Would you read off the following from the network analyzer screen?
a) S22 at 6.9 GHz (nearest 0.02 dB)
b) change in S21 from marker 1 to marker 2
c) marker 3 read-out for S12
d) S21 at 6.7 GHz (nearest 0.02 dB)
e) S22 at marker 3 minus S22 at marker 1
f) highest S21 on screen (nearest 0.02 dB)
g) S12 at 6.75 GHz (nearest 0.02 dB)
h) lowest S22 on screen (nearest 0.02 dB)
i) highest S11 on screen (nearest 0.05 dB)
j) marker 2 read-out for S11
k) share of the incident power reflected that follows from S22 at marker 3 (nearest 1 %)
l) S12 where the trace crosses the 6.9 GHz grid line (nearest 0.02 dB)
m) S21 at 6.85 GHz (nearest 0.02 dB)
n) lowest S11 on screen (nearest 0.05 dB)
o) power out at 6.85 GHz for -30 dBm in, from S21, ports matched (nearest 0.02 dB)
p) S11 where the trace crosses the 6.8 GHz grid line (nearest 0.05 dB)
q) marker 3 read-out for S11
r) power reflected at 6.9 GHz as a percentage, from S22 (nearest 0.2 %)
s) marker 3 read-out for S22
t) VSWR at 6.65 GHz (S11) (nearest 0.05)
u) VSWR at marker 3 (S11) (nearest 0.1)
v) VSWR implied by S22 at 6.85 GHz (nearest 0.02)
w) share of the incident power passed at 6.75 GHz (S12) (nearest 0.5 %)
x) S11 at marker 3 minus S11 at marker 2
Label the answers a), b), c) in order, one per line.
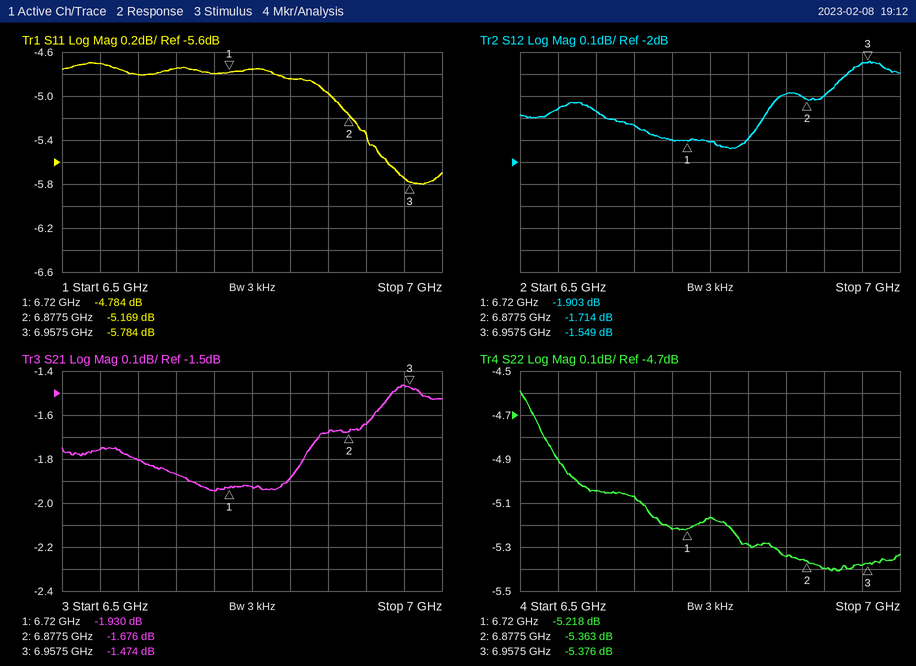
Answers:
a) -5.40 dB
b) 0.254 dB
c) -1.549 dB
d) -1.94 dB
e) -0.158 dB
f) -1.46 dB
g) -1.90 dB
h) -5.40 dB
i) -4.70 dB
j) -5.169 dB
k) 29 %
l) -1.70 dB
m) -1.68 dB
n) -5.80 dB
o) -31.68 dBm
p) -4.85 dB
q) -5.784 dB
r) 28.8 %
s) -5.376 dB
t) 3.75
u) 3.1
v) 3.36
w) 64.5 %
x) -0.615 dB
